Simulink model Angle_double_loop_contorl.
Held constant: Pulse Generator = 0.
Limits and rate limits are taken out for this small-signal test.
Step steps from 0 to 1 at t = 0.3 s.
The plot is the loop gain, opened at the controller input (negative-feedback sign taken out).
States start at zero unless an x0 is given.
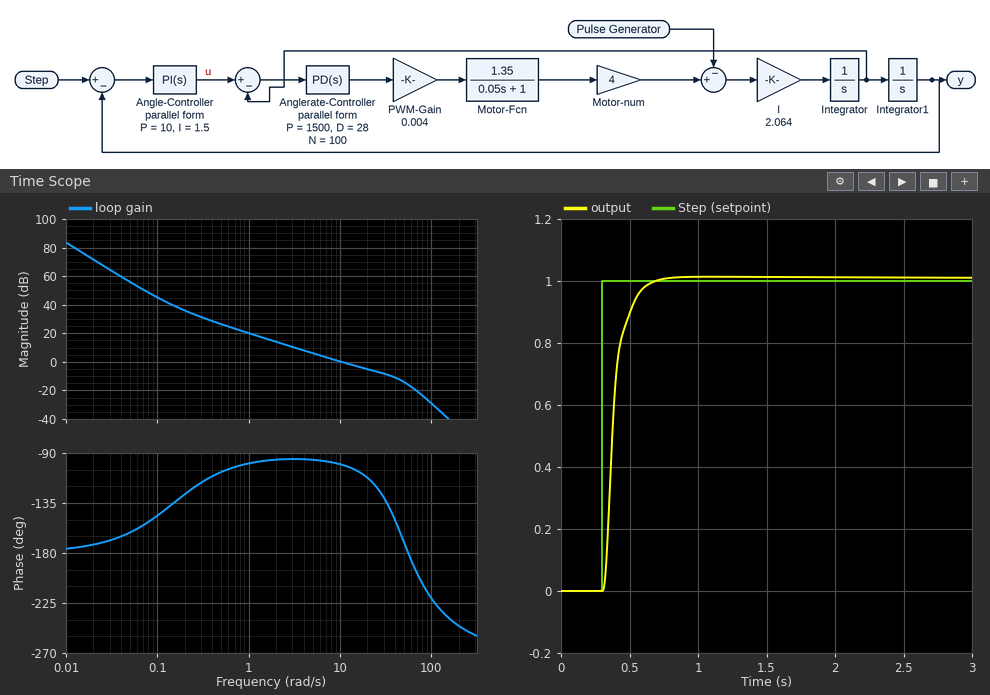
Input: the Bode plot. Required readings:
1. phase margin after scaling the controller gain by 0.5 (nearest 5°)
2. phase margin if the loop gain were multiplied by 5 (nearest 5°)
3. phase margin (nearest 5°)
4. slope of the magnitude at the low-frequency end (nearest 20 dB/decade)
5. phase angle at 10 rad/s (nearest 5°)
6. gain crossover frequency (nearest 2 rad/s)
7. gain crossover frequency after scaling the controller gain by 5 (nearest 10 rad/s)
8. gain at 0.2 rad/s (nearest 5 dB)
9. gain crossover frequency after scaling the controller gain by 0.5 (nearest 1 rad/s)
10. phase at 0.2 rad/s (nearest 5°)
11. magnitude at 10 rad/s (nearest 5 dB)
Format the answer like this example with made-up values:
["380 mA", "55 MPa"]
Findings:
["85°", "10°", "80°", "-40 dB/decade", "-100°", "10 rad/s", "50 rad/s", "35 dB", "5 rad/s", "-125°", "0 dB"]
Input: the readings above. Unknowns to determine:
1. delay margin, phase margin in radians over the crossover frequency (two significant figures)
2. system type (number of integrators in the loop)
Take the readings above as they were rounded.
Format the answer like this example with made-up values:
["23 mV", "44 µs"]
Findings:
["0.14 s", "2"]
